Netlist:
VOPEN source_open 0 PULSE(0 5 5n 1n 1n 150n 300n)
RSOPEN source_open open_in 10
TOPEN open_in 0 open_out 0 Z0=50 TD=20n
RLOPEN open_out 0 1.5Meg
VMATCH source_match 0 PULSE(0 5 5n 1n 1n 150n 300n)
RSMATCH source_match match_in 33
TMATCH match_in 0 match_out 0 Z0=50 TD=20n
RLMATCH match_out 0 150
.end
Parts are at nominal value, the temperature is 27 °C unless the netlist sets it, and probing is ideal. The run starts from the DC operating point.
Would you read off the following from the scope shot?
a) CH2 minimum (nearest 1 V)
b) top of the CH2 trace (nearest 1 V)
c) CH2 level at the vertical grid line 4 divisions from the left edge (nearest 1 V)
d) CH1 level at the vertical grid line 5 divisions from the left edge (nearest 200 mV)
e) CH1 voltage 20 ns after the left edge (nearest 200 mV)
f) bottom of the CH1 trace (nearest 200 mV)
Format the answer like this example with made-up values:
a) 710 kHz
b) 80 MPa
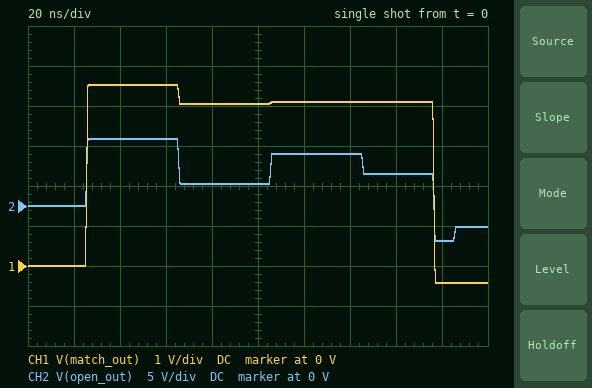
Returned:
a) -4 V
b) 8 V
c) 3 V
d) 4.0 V
e) 0 V
f) -400 mV
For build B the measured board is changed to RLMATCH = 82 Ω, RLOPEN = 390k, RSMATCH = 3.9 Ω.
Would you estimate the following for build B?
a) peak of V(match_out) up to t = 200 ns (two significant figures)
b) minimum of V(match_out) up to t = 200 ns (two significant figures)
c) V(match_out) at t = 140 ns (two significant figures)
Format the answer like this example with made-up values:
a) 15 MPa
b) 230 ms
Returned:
a) 5.8 V
b) -1.0 V
c) 4.8 V
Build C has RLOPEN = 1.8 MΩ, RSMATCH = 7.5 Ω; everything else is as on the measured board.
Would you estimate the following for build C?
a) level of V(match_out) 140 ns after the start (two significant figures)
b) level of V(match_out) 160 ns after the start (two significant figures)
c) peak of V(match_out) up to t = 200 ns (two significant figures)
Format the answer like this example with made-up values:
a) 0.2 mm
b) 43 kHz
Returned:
a) 5.0 V
b) 4.7 V
c) 6.5 V
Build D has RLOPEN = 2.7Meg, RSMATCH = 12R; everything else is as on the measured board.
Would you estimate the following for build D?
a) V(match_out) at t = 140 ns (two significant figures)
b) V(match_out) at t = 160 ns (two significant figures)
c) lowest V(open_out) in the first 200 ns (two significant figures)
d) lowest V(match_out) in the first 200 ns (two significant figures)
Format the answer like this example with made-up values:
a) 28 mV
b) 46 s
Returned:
a) 4.8 V
b) 4.6 V
c) -4.3 V
d) -1.5 V
